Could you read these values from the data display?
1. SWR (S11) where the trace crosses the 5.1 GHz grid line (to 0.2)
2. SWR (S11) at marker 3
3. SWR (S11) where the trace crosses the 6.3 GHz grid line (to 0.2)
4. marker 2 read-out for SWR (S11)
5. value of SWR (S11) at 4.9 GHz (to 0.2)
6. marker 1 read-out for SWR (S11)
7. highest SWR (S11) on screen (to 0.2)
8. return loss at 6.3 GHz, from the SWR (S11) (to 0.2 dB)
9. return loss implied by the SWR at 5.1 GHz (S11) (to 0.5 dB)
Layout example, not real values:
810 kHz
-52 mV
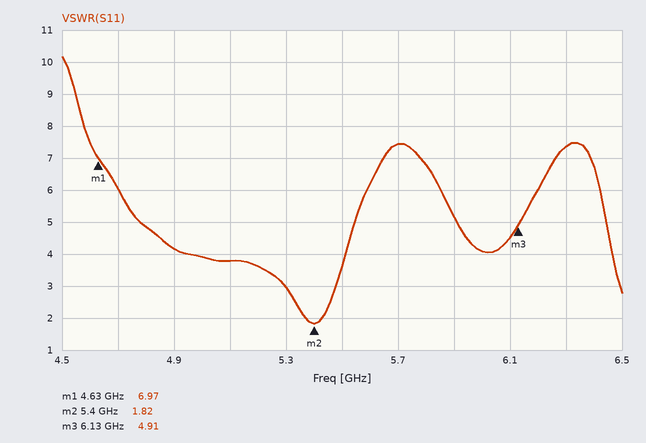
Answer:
3.8
4.91
7.4
1.82
4.2
6.97
10.2
2.4 dB
4.5 dB
